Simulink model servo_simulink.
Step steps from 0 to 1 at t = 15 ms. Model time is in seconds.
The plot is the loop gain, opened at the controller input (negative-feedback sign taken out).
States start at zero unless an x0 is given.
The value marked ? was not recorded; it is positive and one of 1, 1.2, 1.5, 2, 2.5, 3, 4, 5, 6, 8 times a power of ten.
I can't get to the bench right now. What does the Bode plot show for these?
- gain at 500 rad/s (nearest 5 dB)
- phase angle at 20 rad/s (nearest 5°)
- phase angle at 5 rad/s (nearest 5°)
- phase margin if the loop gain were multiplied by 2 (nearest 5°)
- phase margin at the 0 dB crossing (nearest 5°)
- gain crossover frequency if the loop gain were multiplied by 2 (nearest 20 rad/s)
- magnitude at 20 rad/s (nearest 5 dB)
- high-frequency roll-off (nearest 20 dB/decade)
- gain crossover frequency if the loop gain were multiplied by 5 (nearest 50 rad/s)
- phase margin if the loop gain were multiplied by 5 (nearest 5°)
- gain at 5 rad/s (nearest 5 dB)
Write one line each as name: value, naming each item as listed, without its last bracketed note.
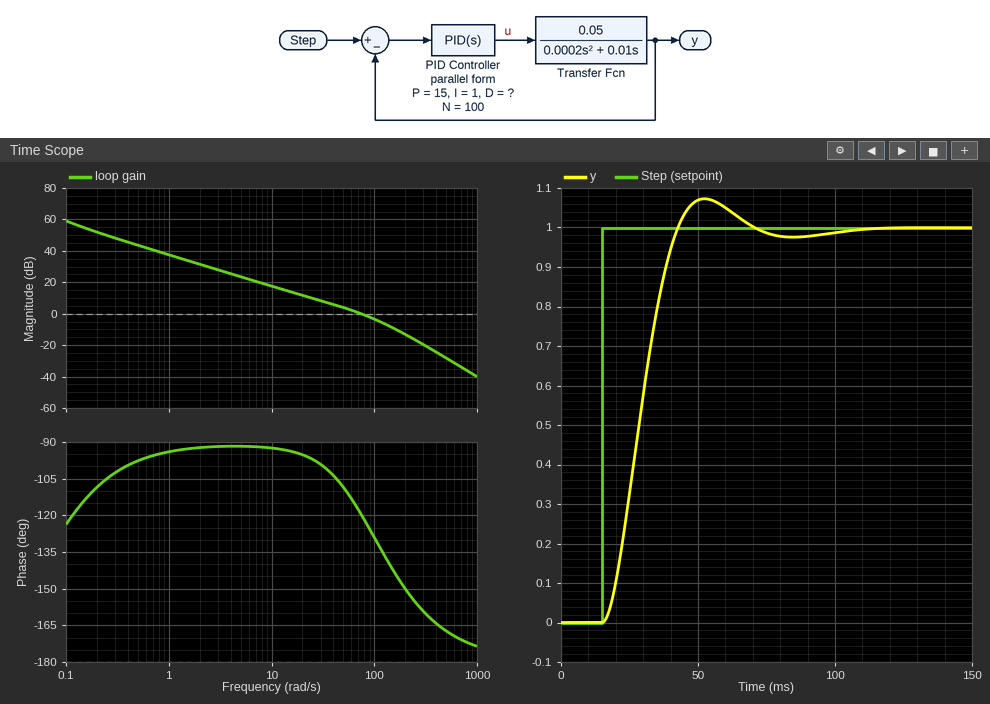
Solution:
gain at 500 rad/s: -30 dB
phase angle at 20 rad/s: -95°
phase angle at 5 rad/s: -90°
phase margin if the loop gain were multiplied by 2: 45°
phase margin at the 0 dB crossing: 60°
gain crossover frequency if the loop gain were multiplied by 2: 120 rad/s
magnitude at 20 rad/s: 10 dB
high-frequency roll-off: -40 dB/decade
gain crossover frequency if the loop gain were multiplied by 5: 200 rad/s
phase margin if the loop gain were multiplied by 5: 30°
gain at 5 rad/s: 25 dB
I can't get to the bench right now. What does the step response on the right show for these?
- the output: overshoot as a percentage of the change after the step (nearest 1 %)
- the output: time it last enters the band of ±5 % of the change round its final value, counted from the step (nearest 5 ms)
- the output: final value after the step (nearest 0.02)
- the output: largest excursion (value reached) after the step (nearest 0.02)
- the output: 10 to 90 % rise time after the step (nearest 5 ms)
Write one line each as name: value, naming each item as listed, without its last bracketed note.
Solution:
the output: overshoot as a percentage of the change after the step: 7 %
the output: time it last enters the band of ±5 % of the change round its final value, counted from the step: 45 ms
the output: final value after the step: 1.00
the output: largest excursion (value reached) after the step: 1.08
the output: 10 to 90 % rise time after the step: 20 ms
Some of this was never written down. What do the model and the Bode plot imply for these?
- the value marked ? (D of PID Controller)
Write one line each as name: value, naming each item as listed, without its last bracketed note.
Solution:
the value marked ?: 0.25
